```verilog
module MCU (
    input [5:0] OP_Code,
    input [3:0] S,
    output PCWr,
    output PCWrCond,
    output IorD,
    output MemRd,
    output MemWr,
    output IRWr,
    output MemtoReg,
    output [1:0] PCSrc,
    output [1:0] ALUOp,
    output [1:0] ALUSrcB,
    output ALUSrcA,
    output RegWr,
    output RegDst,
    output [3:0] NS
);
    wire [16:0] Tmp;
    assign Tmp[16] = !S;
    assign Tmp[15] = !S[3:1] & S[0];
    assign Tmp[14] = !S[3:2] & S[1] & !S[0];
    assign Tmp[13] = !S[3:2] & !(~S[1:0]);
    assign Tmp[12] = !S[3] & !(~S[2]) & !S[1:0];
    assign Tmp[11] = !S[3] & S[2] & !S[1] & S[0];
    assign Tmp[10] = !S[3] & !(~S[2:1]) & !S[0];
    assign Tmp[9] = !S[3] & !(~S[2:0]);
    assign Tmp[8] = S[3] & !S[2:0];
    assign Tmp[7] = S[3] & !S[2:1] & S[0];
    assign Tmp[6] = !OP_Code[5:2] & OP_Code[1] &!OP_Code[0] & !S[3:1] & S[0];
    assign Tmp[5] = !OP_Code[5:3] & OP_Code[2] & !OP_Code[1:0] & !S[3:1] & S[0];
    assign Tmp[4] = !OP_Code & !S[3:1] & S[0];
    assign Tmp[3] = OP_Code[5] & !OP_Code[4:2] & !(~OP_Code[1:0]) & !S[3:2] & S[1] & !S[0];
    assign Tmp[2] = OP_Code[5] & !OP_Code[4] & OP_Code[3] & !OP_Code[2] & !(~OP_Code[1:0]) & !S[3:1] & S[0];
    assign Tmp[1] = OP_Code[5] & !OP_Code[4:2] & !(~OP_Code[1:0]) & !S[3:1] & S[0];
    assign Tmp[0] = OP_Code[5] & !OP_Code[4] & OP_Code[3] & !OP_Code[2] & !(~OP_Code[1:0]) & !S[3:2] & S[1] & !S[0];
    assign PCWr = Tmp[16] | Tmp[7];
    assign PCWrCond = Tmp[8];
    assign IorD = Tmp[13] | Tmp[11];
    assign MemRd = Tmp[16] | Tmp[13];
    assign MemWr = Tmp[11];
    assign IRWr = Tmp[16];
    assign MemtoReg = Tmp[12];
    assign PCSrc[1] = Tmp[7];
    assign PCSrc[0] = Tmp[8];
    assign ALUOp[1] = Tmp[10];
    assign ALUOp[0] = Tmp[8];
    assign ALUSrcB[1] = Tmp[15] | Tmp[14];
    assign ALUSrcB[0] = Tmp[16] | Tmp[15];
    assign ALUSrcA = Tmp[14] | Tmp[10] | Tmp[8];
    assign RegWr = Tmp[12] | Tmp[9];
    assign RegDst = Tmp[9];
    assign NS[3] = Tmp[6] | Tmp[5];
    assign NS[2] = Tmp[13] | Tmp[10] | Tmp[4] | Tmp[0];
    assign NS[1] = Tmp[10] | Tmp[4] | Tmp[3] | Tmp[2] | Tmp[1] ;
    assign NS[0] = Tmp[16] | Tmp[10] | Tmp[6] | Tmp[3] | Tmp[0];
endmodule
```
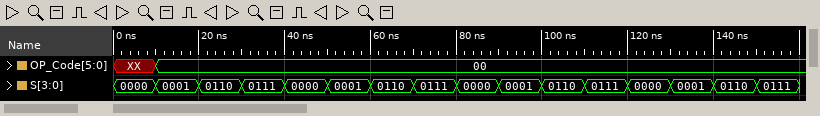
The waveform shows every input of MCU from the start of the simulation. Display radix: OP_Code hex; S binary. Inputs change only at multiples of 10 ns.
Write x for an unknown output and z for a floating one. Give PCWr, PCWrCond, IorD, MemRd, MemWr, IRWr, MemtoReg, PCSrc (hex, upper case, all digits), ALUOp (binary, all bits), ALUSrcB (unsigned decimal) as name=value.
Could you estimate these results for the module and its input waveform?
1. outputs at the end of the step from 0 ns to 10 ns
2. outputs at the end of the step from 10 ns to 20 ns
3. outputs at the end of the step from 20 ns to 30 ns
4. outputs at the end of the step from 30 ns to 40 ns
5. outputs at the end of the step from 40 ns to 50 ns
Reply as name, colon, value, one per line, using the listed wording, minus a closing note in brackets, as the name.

outputs at the end of the step from 0 ns to 10 ns: PCWr=1, PCWrCond=0, IorD=0, MemRd=1, MemWr=0, IRWr=1, MemtoReg=0, PCSrc=0, ALUOp=00, ALUSrcB=1
outputs at the end of the step from 10 ns to 20 ns: PCWr=0, PCWrCond=0, IorD=0, MemRd=0, MemWr=0, IRWr=0, MemtoReg=0, PCSrc=0, ALUOp=00, ALUSrcB=3
outputs at the end of the step from 20 ns to 30 ns: PCWr=0, PCWrCond=0, IorD=0, MemRd=0, MemWr=0, IRWr=0, MemtoReg=0, PCSrc=0, ALUOp=10, ALUSrcB=0
outputs at the end of the step from 30 ns to 40 ns: PCWr=0, PCWrCond=0, IorD=0, MemRd=0, MemWr=0, IRWr=0, MemtoReg=0, PCSrc=0, ALUOp=00, ALUSrcB=0
outputs at the end of the step from 40 ns to 50 ns: PCWr=1, PCWrCond=0, IorD=0, MemRd=1, MemWr=0, IRWr=1, MemtoReg=0, PCSrc=0, ALUOp=00, ALUSrcB=1
